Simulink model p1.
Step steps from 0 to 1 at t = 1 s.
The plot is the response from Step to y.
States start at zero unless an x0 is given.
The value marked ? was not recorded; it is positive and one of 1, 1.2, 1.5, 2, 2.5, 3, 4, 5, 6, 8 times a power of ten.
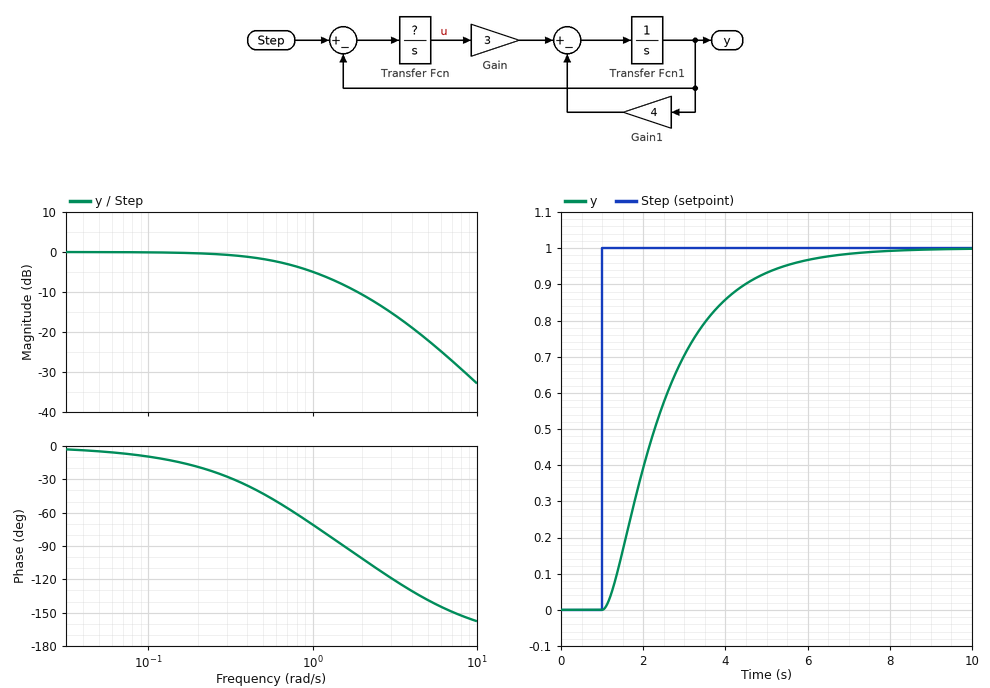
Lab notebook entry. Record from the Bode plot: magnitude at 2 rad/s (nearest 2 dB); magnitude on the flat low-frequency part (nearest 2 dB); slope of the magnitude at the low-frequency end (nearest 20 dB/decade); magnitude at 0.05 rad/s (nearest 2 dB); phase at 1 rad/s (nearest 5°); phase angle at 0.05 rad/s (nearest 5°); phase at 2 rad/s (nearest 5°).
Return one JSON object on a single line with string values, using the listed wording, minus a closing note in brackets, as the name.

{"magnitude at 2 rad/s": "-10 dB", "magnitude on the flat low-frequency part": "0 dB", "slope of the magnitude at the low-frequency end": "0 dB/decade", "magnitude at 0.05 rad/s": "0 dB", "phase at 1 rad/s": "-70°", "phase angle at 0.05 rad/s": "-5°", "phase at 2 rad/s": "-100°"}
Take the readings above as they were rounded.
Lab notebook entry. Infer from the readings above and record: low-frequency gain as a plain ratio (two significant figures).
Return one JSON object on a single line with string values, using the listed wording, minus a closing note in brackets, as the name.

{"low-frequency gain as a plain ratio": "1.0"}
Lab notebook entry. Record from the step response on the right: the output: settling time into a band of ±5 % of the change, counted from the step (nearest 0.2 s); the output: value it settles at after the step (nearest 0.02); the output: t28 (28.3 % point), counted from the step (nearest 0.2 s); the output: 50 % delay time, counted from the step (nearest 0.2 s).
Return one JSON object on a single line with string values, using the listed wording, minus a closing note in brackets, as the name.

{"the output: settling time into a band of ±5 % of the change, counted from the step": "4.4 s", "the output: value it settles at after the step": "1.00", "the output: t28 (28.3 % point), counted from the step": "0.8 s", "the output: 50 % delay time, counted from the step": "1.2 s"}
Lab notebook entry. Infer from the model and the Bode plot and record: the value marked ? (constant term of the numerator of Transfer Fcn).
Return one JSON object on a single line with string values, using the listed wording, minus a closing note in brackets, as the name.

{"the value marked ?": "0.8"}
